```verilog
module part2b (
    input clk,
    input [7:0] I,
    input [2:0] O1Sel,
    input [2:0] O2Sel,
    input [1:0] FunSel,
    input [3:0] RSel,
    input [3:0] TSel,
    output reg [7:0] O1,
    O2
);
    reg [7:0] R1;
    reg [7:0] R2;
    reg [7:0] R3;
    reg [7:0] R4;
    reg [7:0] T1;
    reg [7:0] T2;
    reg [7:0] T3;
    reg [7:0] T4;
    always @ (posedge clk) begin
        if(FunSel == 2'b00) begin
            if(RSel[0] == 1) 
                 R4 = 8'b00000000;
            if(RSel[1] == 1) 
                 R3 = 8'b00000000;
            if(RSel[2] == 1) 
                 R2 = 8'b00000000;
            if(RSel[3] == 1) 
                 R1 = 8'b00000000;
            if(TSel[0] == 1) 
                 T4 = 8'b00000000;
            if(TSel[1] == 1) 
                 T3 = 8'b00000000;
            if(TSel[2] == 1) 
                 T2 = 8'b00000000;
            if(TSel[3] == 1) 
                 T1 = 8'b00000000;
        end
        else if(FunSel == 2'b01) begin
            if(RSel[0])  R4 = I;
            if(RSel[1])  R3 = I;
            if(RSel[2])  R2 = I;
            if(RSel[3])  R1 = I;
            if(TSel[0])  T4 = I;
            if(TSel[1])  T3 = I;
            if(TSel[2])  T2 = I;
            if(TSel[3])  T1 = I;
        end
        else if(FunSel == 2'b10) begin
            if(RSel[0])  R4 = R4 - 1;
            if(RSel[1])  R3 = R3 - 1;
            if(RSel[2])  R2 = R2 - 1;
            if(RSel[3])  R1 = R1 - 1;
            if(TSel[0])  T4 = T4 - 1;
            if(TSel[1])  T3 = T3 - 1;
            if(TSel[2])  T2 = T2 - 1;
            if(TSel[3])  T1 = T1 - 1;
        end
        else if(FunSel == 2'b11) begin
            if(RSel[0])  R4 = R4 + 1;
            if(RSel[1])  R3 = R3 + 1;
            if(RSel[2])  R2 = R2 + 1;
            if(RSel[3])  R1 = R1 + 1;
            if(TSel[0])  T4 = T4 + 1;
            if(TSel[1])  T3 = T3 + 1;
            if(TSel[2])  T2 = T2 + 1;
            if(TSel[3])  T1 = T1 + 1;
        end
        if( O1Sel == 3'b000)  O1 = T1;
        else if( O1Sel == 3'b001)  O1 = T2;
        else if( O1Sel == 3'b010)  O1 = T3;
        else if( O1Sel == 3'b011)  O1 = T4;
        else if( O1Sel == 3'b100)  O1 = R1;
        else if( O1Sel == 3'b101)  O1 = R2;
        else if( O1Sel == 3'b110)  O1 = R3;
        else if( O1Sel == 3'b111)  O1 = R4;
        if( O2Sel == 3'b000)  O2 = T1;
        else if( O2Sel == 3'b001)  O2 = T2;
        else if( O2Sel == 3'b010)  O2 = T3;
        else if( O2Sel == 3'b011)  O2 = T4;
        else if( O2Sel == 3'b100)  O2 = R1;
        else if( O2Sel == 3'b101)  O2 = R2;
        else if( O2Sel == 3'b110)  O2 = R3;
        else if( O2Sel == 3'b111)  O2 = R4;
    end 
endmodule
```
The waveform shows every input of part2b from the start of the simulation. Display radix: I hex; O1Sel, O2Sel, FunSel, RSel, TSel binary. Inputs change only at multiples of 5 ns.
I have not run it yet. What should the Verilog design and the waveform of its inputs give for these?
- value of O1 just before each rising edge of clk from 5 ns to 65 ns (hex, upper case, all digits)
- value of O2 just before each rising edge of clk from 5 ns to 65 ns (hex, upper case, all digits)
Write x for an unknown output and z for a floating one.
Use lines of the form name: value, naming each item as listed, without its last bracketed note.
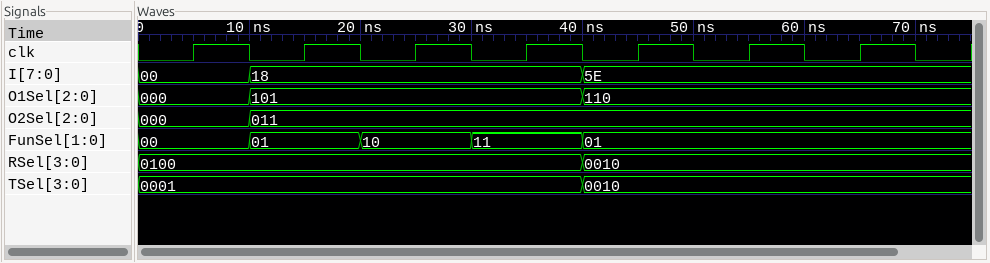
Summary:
value of O1 just before each rising edge of clk from 5 ns to 65 ns: x, x, 18, 17, 18, 5E, 5E
value of O2 just before each rising edge of clk from 5 ns to 65 ns: x, x, 18, 17, 18, 18, 18
